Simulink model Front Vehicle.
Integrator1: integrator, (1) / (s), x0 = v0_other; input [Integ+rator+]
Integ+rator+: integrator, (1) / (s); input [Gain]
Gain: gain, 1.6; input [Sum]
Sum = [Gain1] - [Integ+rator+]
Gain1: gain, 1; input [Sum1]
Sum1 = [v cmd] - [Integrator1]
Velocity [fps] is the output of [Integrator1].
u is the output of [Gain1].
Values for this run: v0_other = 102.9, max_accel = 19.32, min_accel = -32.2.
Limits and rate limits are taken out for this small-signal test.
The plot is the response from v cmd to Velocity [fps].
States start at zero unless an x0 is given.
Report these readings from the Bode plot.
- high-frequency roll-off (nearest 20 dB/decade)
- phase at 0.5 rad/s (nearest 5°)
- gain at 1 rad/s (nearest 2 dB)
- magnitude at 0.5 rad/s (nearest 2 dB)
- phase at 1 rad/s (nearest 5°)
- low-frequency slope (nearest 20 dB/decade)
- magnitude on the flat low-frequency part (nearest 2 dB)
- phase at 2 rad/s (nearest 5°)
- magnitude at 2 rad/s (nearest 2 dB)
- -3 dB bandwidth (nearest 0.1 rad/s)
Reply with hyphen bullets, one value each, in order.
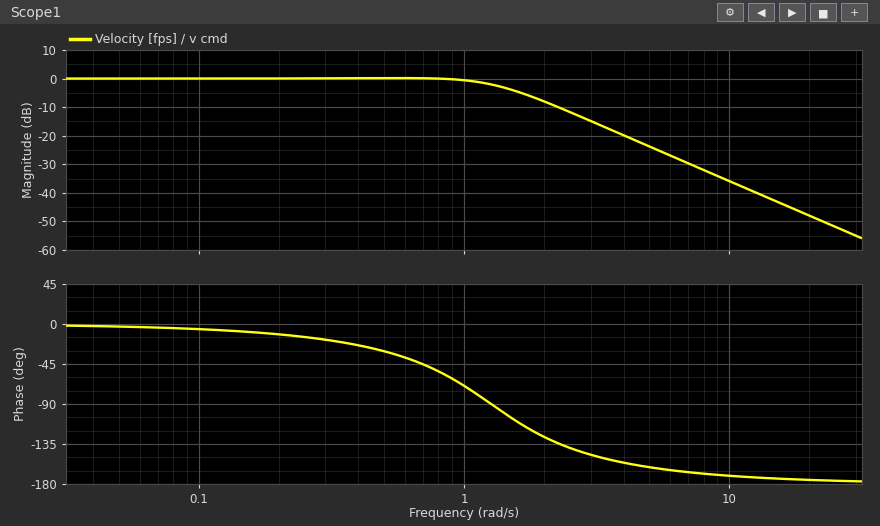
- -40 dB/decade
- -30°
- 0 dB
- 0 dB
- -70°
- 0 dB/decade
- 0 dB
- -125°
- -8 dB
- 1.4 rad/s
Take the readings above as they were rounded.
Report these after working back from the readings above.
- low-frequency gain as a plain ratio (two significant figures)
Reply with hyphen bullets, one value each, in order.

- 1.0
